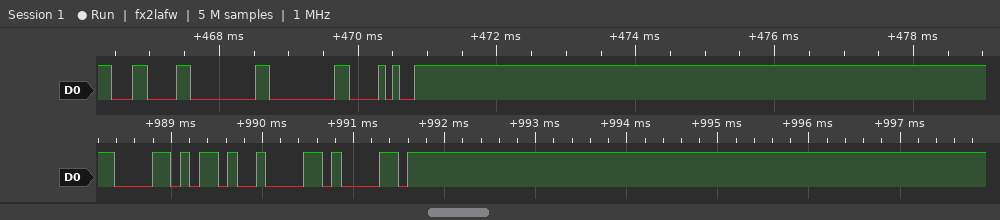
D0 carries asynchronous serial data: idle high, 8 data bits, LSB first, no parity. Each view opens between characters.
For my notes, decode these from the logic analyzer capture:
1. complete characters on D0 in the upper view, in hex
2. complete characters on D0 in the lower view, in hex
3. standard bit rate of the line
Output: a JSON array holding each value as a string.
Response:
["0C, 00, 00, 28", "58, 09, 61", "9600 baud"]
